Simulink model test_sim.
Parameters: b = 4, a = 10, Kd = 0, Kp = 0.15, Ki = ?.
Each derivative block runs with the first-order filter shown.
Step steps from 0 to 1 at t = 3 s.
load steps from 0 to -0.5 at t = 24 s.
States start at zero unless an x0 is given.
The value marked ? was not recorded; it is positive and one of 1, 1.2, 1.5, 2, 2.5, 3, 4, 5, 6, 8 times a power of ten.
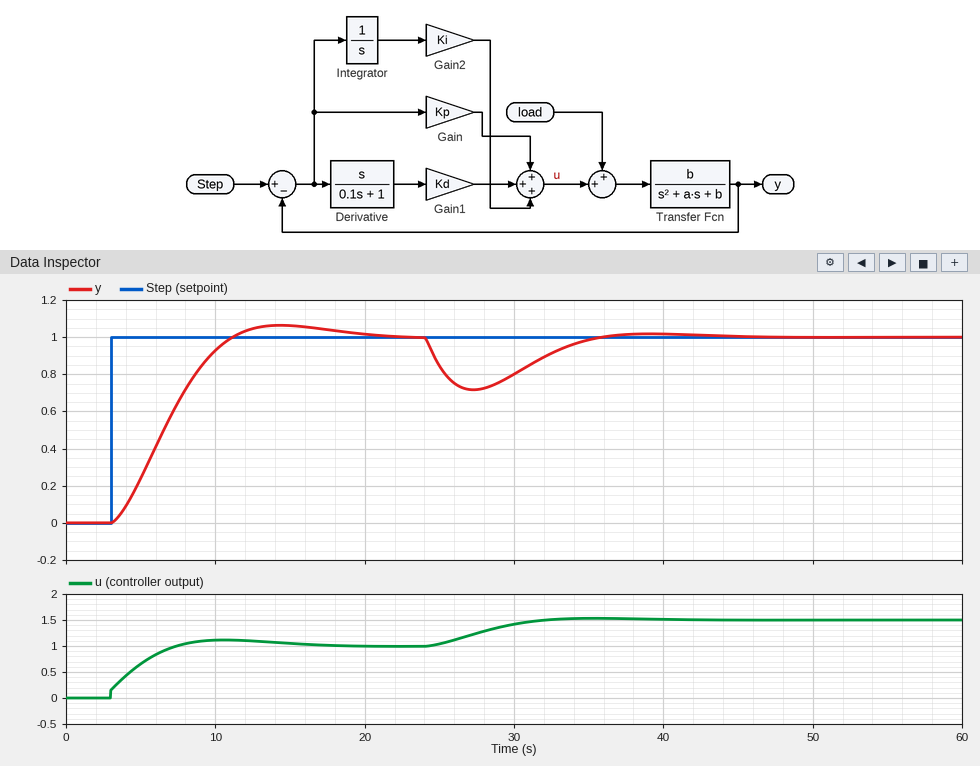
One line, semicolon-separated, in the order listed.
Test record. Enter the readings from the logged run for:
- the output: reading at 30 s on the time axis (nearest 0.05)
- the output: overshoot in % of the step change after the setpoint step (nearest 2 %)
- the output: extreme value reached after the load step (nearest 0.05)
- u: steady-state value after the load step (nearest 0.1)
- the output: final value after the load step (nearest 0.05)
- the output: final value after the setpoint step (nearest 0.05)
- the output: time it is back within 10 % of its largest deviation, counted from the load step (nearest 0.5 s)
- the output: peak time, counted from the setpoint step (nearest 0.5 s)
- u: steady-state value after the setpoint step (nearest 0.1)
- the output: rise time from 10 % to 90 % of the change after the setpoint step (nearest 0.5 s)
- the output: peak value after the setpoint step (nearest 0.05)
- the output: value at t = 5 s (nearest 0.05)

0.80; 6 %; 0.70; 1.5; 1.00; 1.00; 10.5 s; 11.5 s; 1.0; 5.5 s; 1.05; 0.25
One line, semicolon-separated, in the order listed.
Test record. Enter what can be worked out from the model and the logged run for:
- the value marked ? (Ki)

0.3
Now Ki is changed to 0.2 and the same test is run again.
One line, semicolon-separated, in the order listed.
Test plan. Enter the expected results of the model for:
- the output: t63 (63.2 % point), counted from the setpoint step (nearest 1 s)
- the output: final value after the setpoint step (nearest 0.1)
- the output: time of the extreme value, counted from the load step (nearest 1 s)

6 s; 1.0; 4 s
